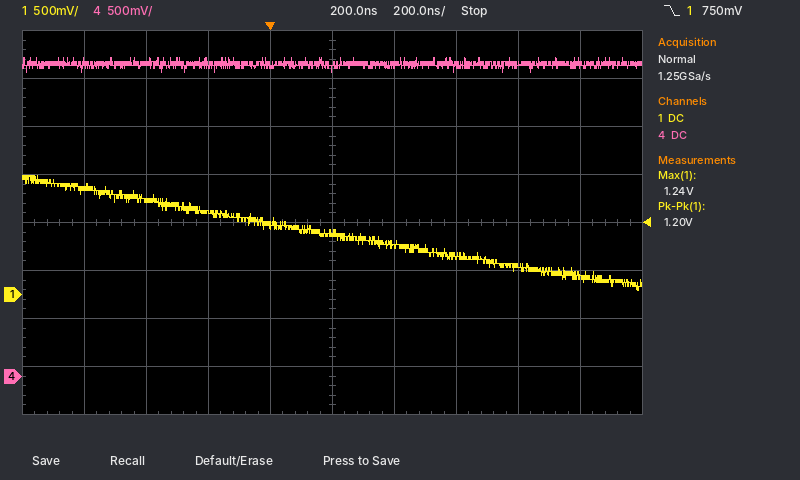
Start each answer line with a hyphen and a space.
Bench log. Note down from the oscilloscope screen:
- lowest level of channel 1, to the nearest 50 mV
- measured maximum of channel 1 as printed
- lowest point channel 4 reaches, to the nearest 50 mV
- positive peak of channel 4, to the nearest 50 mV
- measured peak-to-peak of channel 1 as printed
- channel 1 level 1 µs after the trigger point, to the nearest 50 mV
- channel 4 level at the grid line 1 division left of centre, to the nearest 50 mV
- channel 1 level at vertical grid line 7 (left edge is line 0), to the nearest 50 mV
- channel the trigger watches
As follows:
- 50 mV
- 1.24 V
- 3.15 V
- 3.30 V
- 1.20 V
- 200 mV
- 3.25 V
- 400 mV
- channel 1
